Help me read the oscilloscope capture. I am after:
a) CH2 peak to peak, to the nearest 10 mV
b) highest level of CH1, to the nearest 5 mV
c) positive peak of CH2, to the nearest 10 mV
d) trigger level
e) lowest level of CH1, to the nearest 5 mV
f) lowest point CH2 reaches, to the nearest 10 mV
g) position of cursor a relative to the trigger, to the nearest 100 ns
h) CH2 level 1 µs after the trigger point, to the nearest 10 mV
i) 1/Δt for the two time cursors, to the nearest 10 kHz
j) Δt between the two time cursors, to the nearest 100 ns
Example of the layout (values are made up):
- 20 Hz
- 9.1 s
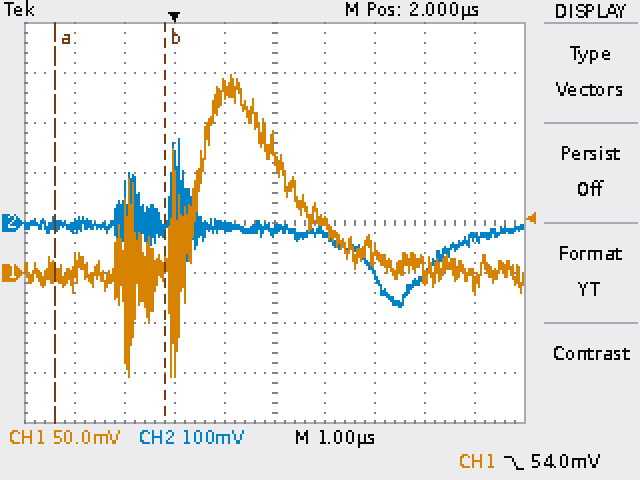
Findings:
- 340 mV
- 200 mV
- 170 mV
- 54.0 mV
- -105 mV
- -170 mV
- -2.4 µs
- -10 mV
- 450 kHz
- 2.2 µs
